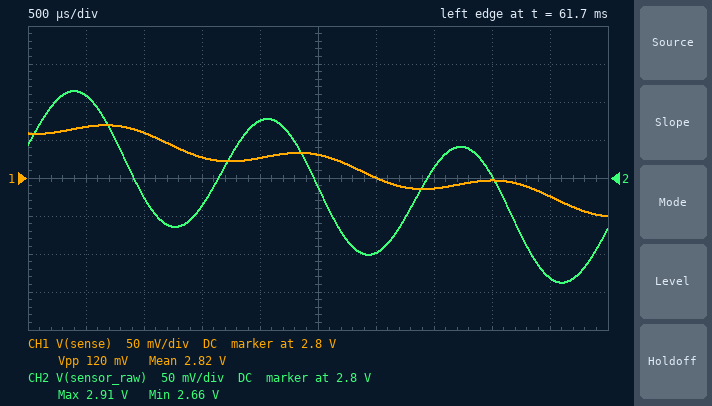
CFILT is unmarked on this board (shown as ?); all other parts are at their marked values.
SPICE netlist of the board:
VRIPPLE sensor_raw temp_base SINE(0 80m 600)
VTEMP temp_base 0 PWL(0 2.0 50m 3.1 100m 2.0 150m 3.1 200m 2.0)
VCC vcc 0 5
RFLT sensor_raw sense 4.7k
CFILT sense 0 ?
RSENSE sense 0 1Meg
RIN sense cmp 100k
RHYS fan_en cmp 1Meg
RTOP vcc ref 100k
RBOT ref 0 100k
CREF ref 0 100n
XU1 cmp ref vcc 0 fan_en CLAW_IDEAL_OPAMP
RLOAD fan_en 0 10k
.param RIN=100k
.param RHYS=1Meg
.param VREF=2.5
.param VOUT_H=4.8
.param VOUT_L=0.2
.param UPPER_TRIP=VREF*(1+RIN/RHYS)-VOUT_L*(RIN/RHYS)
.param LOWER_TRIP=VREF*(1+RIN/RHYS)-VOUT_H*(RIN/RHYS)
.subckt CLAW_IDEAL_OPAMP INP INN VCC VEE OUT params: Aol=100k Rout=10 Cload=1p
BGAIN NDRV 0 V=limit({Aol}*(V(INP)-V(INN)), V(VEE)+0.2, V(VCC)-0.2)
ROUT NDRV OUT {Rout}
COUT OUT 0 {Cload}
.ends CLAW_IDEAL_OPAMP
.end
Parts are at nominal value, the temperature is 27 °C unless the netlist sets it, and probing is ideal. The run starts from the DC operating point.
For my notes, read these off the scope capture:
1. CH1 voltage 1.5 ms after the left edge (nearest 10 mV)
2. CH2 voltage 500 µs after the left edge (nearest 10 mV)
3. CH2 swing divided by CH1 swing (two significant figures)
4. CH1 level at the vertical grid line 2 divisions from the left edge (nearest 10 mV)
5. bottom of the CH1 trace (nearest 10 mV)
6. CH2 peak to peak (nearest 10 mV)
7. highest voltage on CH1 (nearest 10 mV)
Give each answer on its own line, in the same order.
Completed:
2.83 V
2.91 V
2.1
2.86 V
2.75 V
250 mV
2.87 V
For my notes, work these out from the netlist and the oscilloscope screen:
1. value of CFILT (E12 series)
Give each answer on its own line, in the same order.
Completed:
330 nF
